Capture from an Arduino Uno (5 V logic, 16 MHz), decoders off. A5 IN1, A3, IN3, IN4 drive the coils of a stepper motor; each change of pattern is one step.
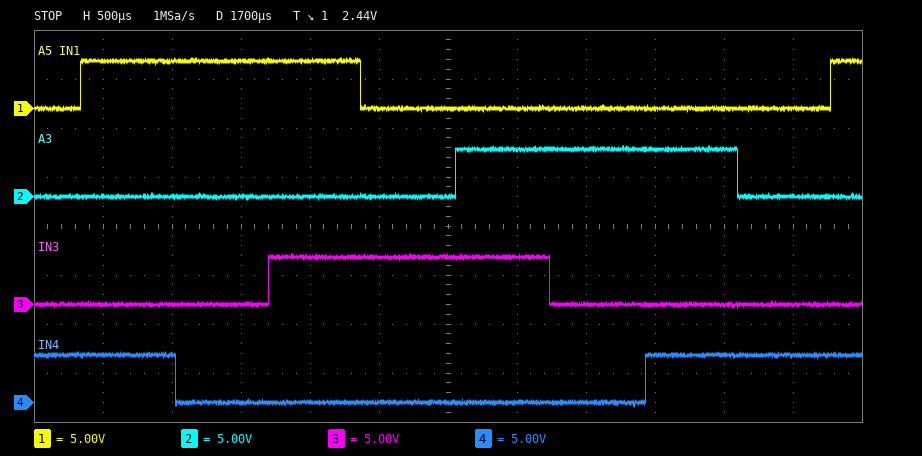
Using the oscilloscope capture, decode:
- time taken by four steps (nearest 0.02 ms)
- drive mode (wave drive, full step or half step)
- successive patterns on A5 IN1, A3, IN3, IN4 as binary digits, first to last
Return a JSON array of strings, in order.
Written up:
["2.72 ms", "half step", "0001 1001 1000 1010 0010 0110 0100 0101 0001 1001"]
